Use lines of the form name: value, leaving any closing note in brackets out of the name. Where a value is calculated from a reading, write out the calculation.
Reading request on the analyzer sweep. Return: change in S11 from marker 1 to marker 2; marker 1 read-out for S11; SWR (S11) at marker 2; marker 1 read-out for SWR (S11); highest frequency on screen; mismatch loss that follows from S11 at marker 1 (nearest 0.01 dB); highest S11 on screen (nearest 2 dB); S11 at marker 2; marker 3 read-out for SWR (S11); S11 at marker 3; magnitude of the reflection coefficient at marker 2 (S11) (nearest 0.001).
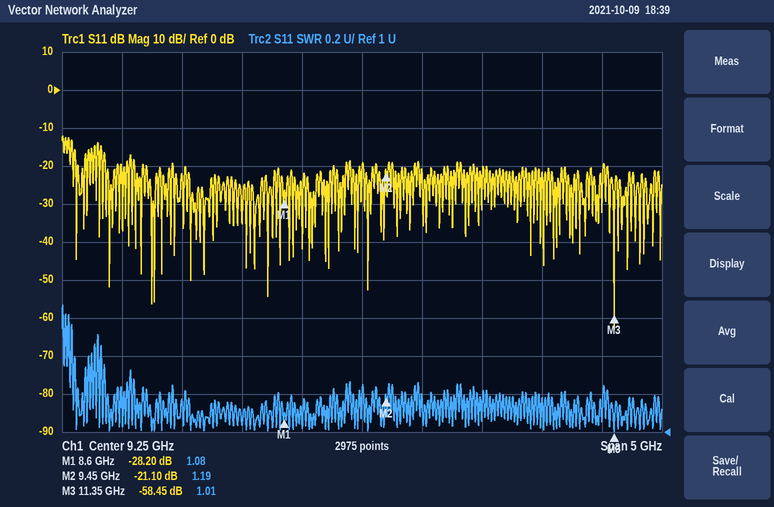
change in S11 from marker 1 to marker 2: -21.1 − (-28.2) = 7.10 dB
marker 1 read-out for S11: -28.20 dB
SWR (S11) at marker 2: 1.19
marker 1 read-out for SWR: 1.08
highest frequency on screen: 11.75 GHz
mismatch loss that follows from S11 at marker 1: −10 log10(1 − 10^(-28.2/10)) ≈ 0.01 dB
highest S11 on screen: -12 dB
S11 at marker 2: -21.10 dB
marker 3 read-out for SWR: 1.01
S11 at marker 3: -58.45 dB
magnitude of the reflection coefficient at marker 2 (S11): 10^(-21.1/20) ≈ 0.088
